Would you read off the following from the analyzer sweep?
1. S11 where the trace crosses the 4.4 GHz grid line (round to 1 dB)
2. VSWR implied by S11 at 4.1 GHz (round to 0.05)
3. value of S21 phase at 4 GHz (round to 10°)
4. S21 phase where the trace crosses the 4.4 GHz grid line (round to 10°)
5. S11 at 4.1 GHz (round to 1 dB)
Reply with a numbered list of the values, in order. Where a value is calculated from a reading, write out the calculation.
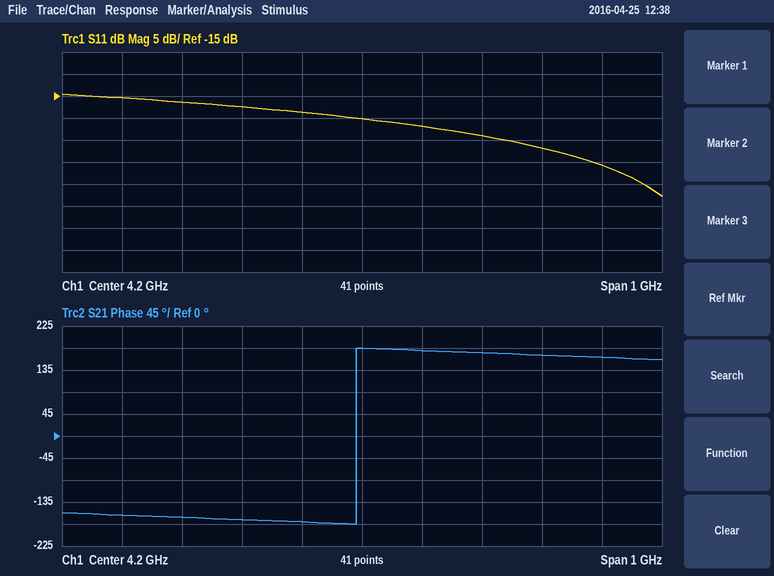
1. -24 dB
2. |Γ| = 10^(-19/20) = 0.1122; VSWR = (1 + 0.1122)/(1 − 0.1122) ≈ 1.25
3. -170°
4. 170°
5. -19 dB
